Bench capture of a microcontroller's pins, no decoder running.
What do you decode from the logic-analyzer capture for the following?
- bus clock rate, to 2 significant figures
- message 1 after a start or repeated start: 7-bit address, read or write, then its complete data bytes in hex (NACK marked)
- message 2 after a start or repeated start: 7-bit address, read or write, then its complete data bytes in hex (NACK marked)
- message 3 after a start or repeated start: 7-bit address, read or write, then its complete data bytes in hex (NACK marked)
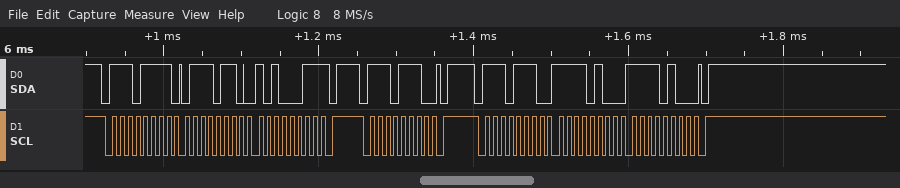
100 kHz
0x77 read: 76 A3 NACK
0x77 write
0x77 write: F4 F4
